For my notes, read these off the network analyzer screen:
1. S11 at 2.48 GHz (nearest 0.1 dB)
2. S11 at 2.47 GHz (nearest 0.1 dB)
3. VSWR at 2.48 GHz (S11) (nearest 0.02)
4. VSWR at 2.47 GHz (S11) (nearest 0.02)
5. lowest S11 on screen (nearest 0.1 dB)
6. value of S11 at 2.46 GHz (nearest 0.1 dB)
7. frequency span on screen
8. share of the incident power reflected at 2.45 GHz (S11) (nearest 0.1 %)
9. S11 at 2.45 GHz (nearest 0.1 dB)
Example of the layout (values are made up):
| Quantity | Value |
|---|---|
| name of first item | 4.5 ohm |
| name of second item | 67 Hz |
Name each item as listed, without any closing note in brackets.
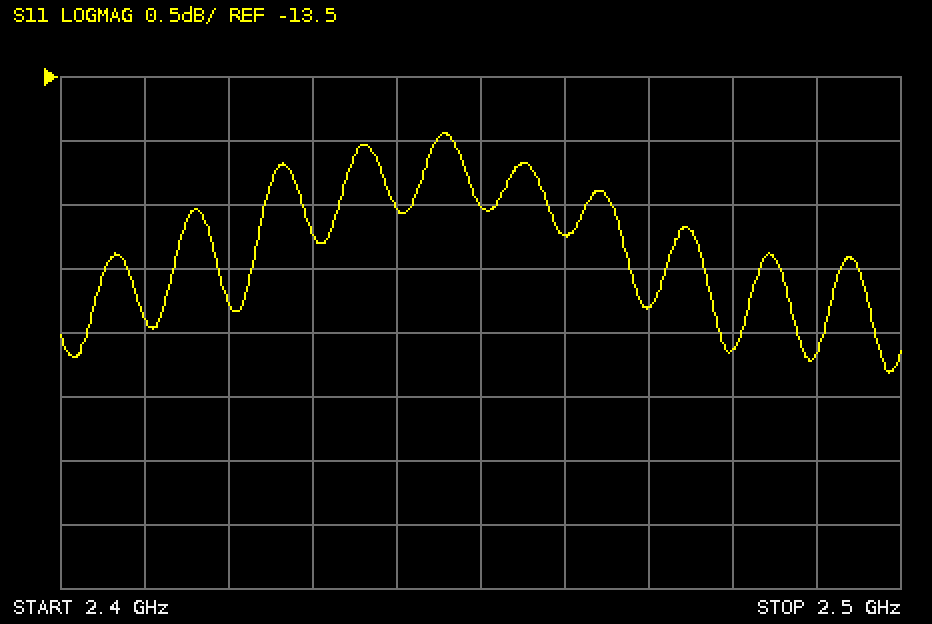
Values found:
| Quantity | Value |
|---|---|
| S11 at 2.48 GHz | -15.6 dB |
| S11 at 2.47 GHz | -15.3 dB |
| VSWR at 2.48 GHz (S11) | 1.40 |
| VSWR at 2.47 GHz (S11) | 1.42 |
| lowest S11 on screen | -15.8 dB |
| value of S11 at 2.46 GHz | -14.7 dB |
| frequency span on screen | 100 MHz |
| share of the incident power reflected at 2.45 GHz (S11) | 3.5 % |
| S11 at 2.45 GHz | -14.5 dB |
